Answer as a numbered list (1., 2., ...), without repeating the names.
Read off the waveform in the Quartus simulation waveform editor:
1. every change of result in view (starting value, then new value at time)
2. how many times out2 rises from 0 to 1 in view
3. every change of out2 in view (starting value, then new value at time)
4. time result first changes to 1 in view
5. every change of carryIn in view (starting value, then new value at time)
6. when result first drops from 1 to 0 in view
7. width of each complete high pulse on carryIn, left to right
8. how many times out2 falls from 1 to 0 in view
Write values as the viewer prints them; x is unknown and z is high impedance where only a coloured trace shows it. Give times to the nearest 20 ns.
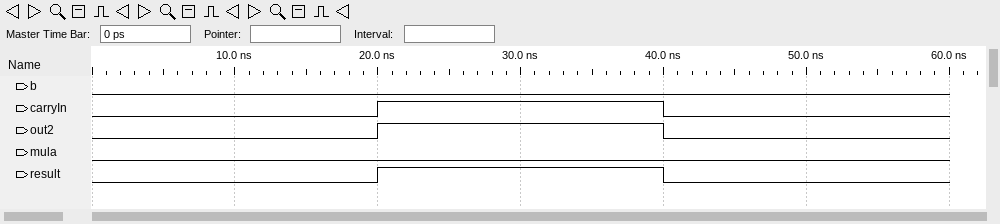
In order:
1. 0, 1 at 20 ns, 0 at 40 ns
2. 1
3. 0, 1 at 20 ns, 0 at 40 ns
4. 20 ns
5. 0, 1 at 20 ns, 0 at 40 ns
6. 40 ns
7. 20 ns
8. 1
